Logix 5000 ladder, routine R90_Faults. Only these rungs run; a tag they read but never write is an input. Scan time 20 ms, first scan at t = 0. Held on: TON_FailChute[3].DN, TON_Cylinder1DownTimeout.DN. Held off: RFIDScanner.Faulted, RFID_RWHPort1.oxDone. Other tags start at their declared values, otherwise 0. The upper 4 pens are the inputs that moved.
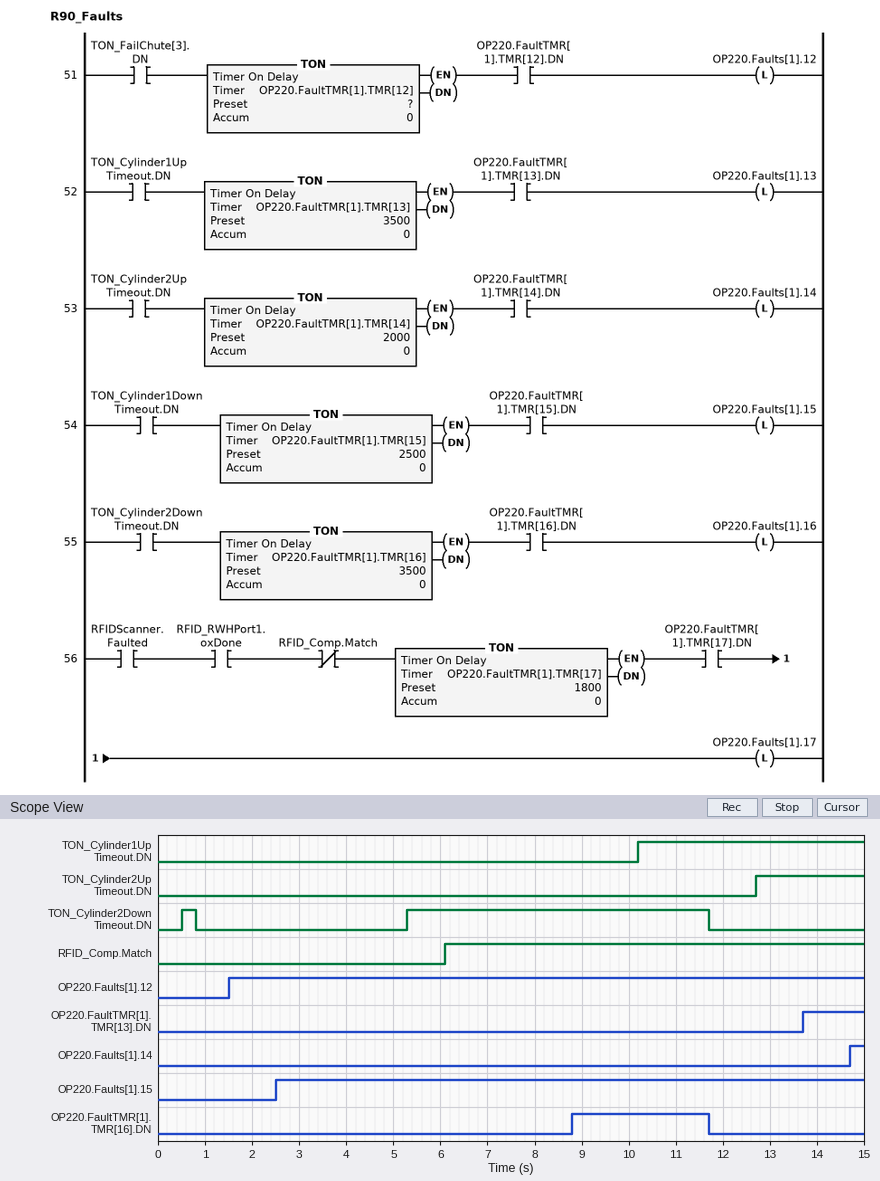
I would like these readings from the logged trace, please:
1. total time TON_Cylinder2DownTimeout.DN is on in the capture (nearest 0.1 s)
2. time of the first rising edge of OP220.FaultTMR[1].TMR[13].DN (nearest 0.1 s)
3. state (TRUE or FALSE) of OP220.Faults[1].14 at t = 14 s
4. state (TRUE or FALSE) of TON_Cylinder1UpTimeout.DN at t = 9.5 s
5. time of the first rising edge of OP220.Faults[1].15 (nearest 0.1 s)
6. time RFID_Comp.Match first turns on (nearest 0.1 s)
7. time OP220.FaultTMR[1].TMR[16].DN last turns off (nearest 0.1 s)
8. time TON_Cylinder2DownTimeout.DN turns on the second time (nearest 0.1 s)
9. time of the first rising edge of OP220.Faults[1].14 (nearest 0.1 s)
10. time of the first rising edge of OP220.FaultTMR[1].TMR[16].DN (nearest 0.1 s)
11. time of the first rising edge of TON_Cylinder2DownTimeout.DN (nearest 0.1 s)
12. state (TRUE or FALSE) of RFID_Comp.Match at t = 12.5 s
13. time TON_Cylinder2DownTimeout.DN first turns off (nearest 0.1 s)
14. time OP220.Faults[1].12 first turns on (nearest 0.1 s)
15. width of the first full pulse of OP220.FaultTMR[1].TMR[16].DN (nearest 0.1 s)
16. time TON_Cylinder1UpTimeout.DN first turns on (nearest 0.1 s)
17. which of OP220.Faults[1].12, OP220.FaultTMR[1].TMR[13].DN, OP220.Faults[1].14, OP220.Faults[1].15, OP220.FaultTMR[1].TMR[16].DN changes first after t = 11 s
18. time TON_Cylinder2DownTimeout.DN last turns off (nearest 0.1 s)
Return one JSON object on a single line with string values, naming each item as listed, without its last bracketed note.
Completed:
{"total time TON_Cylinder2DownTimeout.DN is on in the capture": "6.7 s", "time of the first rising edge of OP220.FaultTMR[1].TMR[13].DN": "13.7 s", "state (TRUE or FALSE) of OP220.Faults[1].14 at t = 14 s": "FALSE", "state (TRUE or FALSE) of TON_Cylinder1UpTimeout.DN at t = 9.5 s": "FALSE", "time of the first rising edge of OP220.Faults[1].15": "2.5 s", "time RFID_Comp.Match first turns on": "6.1 s", "time OP220.FaultTMR[1].TMR[16].DN last turns off": "11.7 s", "time TON_Cylinder2DownTimeout.DN turns on the second time": "5.3 s", "time of the first rising edge of OP220.Faults[1].14": "14.7 s", "time of the first rising edge of OP220.FaultTMR[1].TMR[16].DN": "8.8 s", "time of the first rising edge of TON_Cylinder2DownTimeout.DN": "0.5 s", "state (TRUE or FALSE) of RFID_Comp.Match at t = 12.5 s": "TRUE", "time TON_Cylinder2DownTimeout.DN first turns off": "0.8 s", "time OP220.Faults[1].12 first turns on": "1.5 s", "width of the first full pulse of OP220.FaultTMR[1].TMR[16].DN": "2.9 s", "time TON_Cylinder1UpTimeout.DN first turns on": "10.2 s", "which of OP220.Faults[1].12, OP220.FaultTMR[1].TMR[13].DN, OP220.Faults[1].14, OP220.Faults[1].15, OP220.FaultTMR[1].TMR[16].DN changes first after t = 11 s": "OP220.FaultTMR[1].TMR[16].DN", "time TON_Cylinder2DownTimeout.DN last turns off": "11.7 s"}
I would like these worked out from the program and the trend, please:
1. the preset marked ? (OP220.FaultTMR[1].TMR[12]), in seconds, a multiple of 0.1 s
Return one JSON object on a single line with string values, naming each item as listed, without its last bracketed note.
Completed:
{"the preset marked ? (OP220.FaultTMR[1].TMR[12]), in seconds, a multiple of 0.1 s": "1.5 s"}
